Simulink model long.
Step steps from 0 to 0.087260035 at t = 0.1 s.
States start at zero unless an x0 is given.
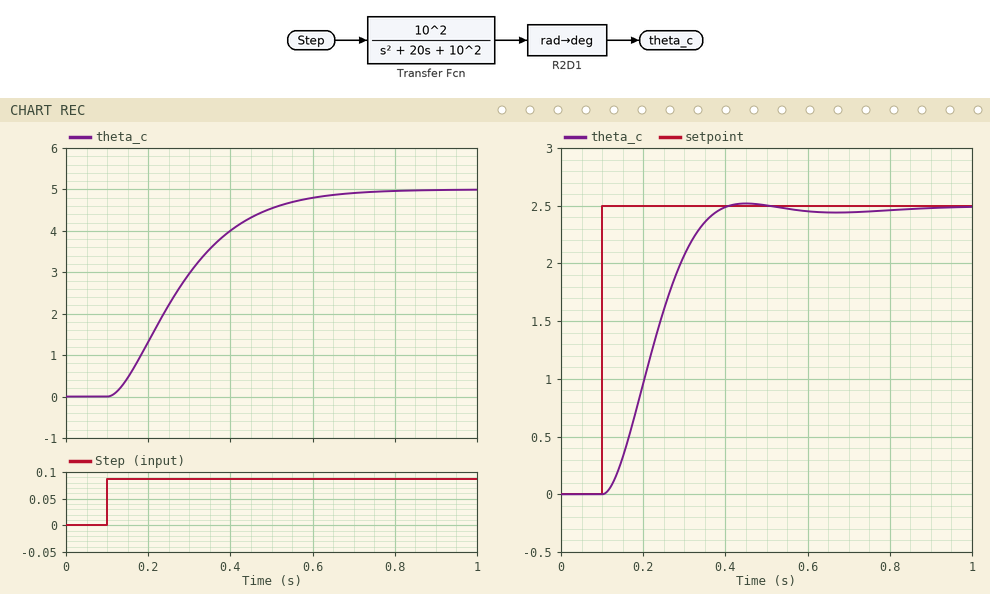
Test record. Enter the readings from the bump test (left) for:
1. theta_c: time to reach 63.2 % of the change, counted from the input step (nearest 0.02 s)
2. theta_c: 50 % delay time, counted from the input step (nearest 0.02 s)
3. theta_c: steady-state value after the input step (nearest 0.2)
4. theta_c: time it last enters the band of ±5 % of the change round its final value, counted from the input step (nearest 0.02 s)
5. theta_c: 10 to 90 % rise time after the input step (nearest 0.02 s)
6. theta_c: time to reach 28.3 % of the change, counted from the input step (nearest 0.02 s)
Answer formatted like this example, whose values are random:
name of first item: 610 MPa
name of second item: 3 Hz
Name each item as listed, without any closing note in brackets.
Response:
theta_c: time to reach 63.2 % of the change, counted from the input step: 0.22 s
theta_c: 50 % delay time, counted from the input step: 0.16 s
theta_c: steady-state value after the input step: 5.0
theta_c: time it last enters the band of ±5 % of the change round its final value, counted from the input step: 0.48 s
theta_c: 10 to 90 % rise time after the input step: 0.34 s
theta_c: time to reach 28.3 % of the change, counted from the input step: 0.10 s
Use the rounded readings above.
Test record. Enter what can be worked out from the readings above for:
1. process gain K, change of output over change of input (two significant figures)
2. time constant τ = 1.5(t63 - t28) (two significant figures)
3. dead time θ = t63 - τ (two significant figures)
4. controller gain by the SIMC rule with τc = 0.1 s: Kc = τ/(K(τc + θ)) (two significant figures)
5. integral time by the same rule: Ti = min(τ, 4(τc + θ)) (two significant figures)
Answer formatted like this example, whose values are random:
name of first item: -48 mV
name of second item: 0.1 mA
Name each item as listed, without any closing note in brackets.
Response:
process gain K, change of output over change of input: 57
time constant τ = 1.5(t63 - t28): 0.18 s
dead time θ = t63 - τ: 0.040 s
controller gain by the SIMC rule with τc = 0.1 s: Kc = τ/(K(τc + θ)): 0.023
integral time by the same rule: Ti = min(τ, 4(τc + θ)): 0.18 s
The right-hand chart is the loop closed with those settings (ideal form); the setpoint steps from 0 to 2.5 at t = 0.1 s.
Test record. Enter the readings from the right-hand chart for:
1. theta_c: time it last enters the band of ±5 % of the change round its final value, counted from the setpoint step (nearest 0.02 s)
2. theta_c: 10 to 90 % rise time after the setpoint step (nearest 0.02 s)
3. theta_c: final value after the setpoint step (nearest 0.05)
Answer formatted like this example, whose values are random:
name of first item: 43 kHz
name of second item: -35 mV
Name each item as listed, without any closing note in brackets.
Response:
theta_c: time it last enters the band of ±5 % of the change round its final value, counted from the setpoint step: 0.26 s
theta_c: 10 to 90 % rise time after the setpoint step: 0.18 s
theta_c: final value after the setpoint step: 2.50
